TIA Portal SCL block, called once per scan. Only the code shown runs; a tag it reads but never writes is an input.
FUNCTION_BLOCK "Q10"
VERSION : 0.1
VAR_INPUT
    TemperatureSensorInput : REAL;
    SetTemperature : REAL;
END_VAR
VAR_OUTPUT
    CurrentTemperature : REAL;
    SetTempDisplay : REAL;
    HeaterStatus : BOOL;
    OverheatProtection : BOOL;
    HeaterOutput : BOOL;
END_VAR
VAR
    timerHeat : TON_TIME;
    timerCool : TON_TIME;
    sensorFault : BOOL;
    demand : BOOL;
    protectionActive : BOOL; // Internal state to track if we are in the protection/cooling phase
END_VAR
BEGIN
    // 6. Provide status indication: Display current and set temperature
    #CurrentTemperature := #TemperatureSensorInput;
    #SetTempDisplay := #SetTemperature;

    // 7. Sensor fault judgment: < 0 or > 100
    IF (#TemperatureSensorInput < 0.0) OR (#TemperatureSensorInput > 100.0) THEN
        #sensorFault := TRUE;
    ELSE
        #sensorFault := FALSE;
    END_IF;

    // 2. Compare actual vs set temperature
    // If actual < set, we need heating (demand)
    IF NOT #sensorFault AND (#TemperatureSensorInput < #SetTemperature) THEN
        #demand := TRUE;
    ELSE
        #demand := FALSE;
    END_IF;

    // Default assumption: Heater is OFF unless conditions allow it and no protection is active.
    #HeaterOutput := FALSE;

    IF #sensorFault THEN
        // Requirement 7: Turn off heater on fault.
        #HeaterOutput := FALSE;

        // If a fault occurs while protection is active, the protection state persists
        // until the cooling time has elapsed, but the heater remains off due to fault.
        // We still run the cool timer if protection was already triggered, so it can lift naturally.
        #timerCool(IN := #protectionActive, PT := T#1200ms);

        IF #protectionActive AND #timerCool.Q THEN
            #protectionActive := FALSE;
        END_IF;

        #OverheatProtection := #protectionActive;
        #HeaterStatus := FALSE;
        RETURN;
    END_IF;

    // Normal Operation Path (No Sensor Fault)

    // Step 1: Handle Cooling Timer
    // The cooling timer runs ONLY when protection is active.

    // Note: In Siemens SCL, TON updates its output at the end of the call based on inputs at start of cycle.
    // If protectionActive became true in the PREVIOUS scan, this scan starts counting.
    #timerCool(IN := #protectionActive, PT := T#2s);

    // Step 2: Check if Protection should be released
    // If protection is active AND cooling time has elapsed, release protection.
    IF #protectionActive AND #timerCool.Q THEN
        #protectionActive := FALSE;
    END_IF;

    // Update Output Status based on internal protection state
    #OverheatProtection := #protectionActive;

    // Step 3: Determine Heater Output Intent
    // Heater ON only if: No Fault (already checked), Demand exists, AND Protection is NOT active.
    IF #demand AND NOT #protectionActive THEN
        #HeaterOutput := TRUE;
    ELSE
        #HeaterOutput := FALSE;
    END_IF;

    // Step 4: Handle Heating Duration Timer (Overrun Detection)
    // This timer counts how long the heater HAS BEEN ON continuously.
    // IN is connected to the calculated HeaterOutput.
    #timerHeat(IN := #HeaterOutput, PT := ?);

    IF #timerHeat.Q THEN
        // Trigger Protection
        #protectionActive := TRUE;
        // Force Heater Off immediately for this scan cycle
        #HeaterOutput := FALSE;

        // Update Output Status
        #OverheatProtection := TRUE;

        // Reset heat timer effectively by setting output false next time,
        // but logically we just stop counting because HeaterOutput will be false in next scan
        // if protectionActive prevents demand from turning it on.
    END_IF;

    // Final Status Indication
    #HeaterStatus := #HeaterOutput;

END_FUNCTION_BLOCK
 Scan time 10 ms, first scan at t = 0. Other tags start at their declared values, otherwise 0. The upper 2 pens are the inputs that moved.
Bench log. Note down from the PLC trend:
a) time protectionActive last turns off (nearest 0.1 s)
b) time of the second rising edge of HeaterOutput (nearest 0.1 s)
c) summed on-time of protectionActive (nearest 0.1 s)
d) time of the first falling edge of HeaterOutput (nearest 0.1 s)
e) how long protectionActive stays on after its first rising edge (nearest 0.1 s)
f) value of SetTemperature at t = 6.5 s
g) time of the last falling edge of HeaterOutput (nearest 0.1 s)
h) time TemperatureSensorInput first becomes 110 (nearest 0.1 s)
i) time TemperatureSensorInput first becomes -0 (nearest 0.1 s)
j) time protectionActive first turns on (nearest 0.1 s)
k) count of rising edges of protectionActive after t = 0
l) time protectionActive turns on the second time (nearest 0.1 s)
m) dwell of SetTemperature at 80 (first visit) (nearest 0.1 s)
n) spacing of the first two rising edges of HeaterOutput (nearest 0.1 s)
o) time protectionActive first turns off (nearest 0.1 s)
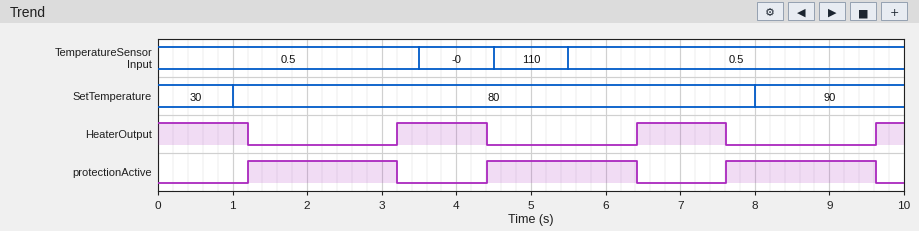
9.6 s
6.4 s
6.0 s
1.2 s
2.0 s
80
7.6 s
4.5 s
3.5 s
1.2 s
3
4.4 s
7.0 s
3.2 s
3.2 s
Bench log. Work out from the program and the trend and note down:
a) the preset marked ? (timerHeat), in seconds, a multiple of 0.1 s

1.2 s
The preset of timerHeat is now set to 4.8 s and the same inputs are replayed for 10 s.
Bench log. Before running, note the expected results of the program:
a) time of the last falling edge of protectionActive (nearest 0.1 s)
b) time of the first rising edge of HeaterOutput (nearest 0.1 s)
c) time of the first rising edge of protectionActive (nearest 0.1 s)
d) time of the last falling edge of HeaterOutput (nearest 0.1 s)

7.5 s
7.5 s
5.5 s
4.5 s
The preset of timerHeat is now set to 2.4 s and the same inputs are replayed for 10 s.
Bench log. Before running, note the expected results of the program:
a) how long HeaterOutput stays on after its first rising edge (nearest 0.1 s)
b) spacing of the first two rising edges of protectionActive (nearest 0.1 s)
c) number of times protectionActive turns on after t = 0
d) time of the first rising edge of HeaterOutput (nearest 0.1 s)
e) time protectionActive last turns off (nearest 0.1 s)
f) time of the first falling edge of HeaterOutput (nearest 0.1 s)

0.1 s
4.4 s
2
4.4 s
8.8 s
2.4 s
